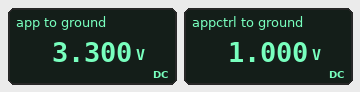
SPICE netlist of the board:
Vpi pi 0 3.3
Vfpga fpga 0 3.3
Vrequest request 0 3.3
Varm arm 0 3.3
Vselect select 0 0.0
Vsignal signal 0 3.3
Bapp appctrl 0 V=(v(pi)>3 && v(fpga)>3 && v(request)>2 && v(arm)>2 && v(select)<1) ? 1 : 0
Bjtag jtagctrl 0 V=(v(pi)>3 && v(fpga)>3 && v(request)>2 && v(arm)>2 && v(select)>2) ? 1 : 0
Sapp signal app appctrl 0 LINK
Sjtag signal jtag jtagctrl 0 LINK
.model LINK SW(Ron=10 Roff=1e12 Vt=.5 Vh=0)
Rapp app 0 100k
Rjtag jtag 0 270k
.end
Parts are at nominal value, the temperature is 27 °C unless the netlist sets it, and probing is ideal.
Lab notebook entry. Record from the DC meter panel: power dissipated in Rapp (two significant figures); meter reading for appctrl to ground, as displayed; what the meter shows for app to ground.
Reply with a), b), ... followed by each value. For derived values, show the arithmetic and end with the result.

a) (3.3 V)^2 / 100 kΩ = 110 µW
b) 1.000 V
c) 3.300 V
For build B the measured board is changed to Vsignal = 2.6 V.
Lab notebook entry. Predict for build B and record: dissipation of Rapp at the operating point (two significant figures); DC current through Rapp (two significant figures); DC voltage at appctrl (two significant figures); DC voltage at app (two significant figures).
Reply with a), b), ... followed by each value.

a) 68 µW
b) 26 µA
c) 1.0 V
d) 2.6 V
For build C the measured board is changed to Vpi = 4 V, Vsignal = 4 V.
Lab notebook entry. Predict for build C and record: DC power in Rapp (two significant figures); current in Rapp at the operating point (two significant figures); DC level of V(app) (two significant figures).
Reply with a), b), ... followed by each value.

a) 160 µW
b) 40 µA
c) 4.0 V
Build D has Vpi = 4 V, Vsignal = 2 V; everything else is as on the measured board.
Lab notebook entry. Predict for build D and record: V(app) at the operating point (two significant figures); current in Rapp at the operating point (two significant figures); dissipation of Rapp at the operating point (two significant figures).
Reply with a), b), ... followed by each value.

a) 2.0 V
b) 20 µA
c) 40 µW
